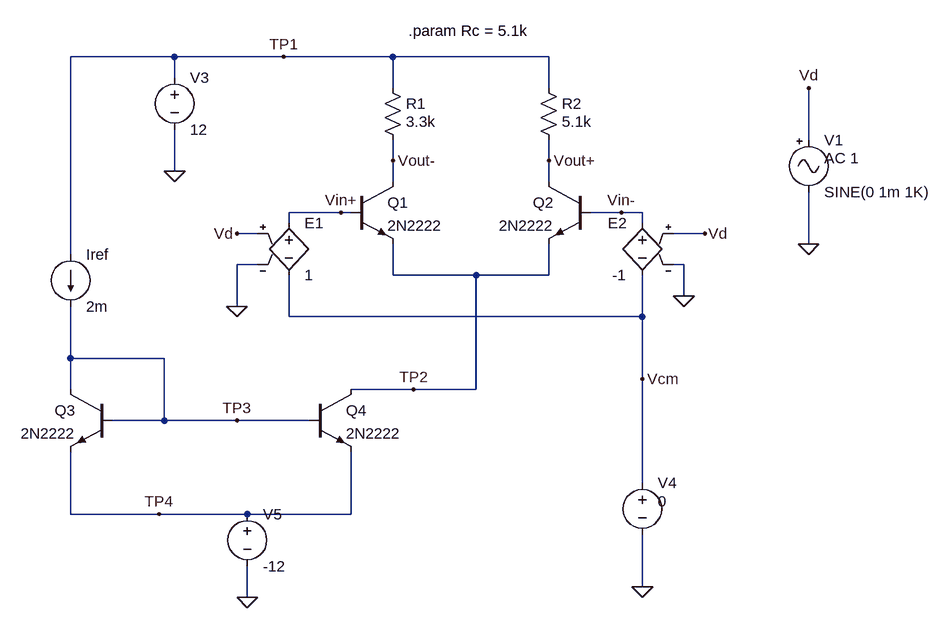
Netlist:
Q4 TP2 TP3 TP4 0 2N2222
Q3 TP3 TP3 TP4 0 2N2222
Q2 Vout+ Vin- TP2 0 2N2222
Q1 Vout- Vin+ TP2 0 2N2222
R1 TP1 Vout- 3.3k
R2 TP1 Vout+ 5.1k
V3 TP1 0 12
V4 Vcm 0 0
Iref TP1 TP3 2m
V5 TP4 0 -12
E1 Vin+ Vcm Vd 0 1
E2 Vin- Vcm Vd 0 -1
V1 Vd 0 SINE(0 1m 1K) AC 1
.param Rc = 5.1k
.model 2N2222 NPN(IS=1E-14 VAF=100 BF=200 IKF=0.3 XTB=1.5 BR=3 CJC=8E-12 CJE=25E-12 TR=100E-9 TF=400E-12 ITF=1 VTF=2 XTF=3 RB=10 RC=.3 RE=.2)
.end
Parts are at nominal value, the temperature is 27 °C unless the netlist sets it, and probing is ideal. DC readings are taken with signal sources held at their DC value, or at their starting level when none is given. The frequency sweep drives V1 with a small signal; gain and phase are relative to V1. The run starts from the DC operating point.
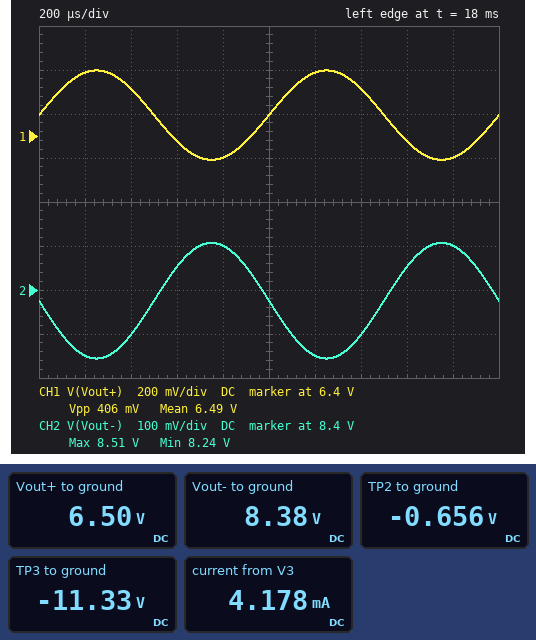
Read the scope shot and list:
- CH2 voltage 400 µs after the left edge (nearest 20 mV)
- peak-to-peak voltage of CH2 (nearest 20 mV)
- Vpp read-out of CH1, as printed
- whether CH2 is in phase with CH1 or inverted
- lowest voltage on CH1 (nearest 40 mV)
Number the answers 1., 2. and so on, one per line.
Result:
1. 8.30 V
2. 260 mV
3. 406 mV
4. inverted
5. 6.28 V
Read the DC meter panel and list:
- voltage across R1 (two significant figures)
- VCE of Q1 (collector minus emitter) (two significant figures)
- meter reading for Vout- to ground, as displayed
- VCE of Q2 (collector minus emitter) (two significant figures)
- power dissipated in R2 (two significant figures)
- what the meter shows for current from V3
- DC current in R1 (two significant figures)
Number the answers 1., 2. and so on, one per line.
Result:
1. 3.6 V
2. 9.0 V
3. 8.38 V
4. 7.2 V
5. 5.9 mW
6. 4.178 mA
7. 1.1 mA
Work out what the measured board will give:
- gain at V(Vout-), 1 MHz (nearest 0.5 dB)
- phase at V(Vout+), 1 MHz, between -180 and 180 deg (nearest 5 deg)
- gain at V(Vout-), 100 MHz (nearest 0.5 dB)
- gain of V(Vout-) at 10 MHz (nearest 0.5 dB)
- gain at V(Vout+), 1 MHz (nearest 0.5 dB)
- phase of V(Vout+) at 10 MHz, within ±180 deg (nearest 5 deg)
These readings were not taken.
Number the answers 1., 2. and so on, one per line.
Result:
1. 42.5 dB
2. -10 deg
3. 22.0 dB
4. 39.0 dB
5. 46.0 dB
6. -60 deg
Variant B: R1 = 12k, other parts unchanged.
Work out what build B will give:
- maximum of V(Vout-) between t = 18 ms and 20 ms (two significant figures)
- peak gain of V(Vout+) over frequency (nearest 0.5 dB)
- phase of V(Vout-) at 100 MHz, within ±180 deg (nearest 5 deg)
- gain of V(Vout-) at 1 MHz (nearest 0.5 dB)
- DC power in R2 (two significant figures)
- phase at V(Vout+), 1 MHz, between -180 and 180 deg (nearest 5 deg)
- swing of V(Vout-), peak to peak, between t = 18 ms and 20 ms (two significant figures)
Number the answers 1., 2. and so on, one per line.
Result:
1. -170 mV
2. 44.0 dB
3. 40 deg
4. 37.5 dB
5. 6.5 mW
6. 5 deg
7. 400 mV
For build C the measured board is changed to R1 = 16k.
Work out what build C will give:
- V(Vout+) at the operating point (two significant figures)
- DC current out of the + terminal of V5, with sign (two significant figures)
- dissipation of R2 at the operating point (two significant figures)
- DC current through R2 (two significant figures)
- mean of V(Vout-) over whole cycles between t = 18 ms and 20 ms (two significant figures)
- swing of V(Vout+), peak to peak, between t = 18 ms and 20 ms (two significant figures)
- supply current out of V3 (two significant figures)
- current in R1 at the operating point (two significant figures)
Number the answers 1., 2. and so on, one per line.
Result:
1. 5.4 V
2. -4.2 mA
3. 8.5 mW
4. 1.3 mA
5. -620 mV
6. 170 mV
7. 4.1 mA
8. 790 µA
